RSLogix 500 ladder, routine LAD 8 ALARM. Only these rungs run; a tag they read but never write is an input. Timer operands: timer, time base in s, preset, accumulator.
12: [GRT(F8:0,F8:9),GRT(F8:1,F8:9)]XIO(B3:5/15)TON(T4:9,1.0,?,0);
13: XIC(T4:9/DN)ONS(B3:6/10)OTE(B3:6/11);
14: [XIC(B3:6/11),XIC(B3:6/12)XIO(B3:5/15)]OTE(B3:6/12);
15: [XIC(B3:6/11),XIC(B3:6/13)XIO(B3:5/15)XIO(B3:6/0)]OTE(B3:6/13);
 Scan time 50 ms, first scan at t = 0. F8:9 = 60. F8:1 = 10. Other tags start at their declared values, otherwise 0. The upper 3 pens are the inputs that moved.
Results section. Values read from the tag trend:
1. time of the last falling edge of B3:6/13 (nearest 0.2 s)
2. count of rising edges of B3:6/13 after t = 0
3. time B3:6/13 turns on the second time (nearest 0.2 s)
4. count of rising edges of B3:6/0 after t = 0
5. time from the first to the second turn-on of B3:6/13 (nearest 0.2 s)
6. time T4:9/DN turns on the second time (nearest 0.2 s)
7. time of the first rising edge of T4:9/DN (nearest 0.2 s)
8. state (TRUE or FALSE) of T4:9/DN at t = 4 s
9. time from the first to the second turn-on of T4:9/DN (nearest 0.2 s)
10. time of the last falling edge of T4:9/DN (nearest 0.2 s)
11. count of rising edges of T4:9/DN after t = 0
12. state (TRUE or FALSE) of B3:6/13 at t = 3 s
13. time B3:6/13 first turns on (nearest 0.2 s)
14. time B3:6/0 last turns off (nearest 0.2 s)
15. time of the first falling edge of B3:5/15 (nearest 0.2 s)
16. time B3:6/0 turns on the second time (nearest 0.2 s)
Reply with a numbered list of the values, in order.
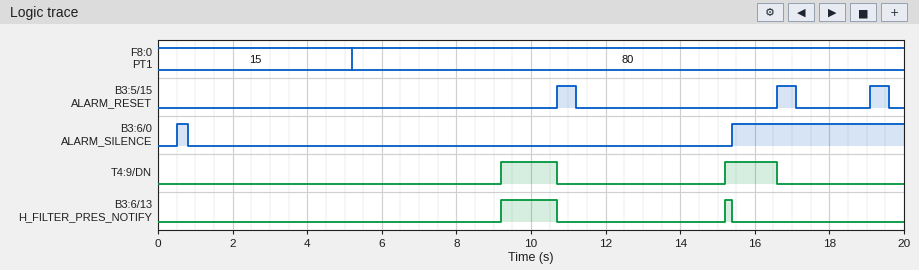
1. 15.4 s
2. 2
3. 15.2 s
4. 2
5. 6.0 s
6. 15.2 s
7. 9.2 s
8. FALSE
9. 6.0 s
10. 16.6 s
11. 2
12. FALSE
13. 9.2 s
14. 0.8 s
15. 11.2 s
16. 15.4 s
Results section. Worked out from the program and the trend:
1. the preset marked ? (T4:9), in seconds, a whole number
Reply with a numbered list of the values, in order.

1. 4 s
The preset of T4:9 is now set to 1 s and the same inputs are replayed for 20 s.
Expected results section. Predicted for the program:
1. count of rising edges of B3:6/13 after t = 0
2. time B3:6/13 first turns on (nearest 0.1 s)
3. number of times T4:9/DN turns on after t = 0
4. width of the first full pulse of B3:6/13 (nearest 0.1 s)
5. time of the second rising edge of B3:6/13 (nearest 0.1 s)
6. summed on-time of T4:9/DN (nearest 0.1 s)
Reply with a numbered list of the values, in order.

1. 3
2. 6.2 s
3. 3
4. 4.5 s
5. 12.2 s
6. 9.9 s
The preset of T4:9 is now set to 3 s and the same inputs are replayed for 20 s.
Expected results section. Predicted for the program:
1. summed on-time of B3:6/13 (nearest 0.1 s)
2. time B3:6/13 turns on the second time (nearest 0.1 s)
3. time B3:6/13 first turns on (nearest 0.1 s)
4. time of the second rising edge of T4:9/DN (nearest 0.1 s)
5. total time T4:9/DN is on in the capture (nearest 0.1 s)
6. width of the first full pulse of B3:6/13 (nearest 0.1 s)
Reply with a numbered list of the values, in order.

1. 3.7 s
2. 14.2 s
3. 8.2 s
4. 14.2 s
5. 4.9 s
6. 2.5 s
